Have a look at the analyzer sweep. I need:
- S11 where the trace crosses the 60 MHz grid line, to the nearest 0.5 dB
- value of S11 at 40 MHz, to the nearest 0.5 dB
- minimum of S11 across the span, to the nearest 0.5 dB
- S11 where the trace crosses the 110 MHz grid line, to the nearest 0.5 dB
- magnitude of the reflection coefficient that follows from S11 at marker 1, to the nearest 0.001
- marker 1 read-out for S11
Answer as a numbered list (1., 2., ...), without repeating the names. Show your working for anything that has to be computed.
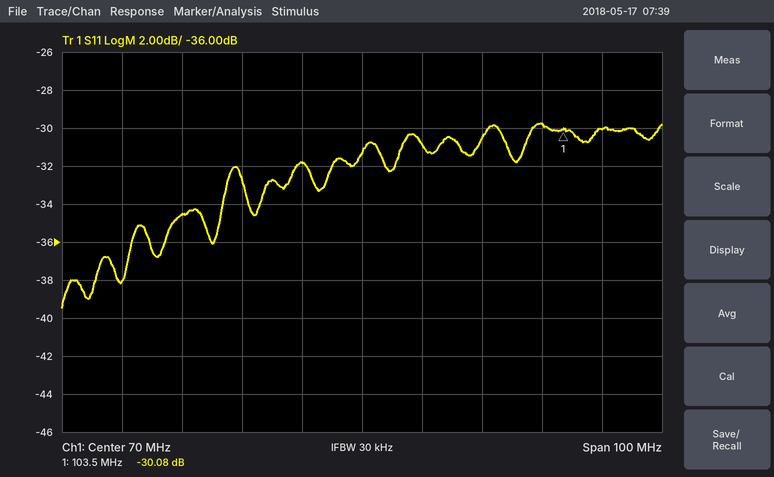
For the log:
1. -32.0 dB
2. -34.5 dB
3. -39.5 dB
4. -30.0 dB
5. 10^(-30.08/20) ≈ 0.031
6. -30.08 dB
